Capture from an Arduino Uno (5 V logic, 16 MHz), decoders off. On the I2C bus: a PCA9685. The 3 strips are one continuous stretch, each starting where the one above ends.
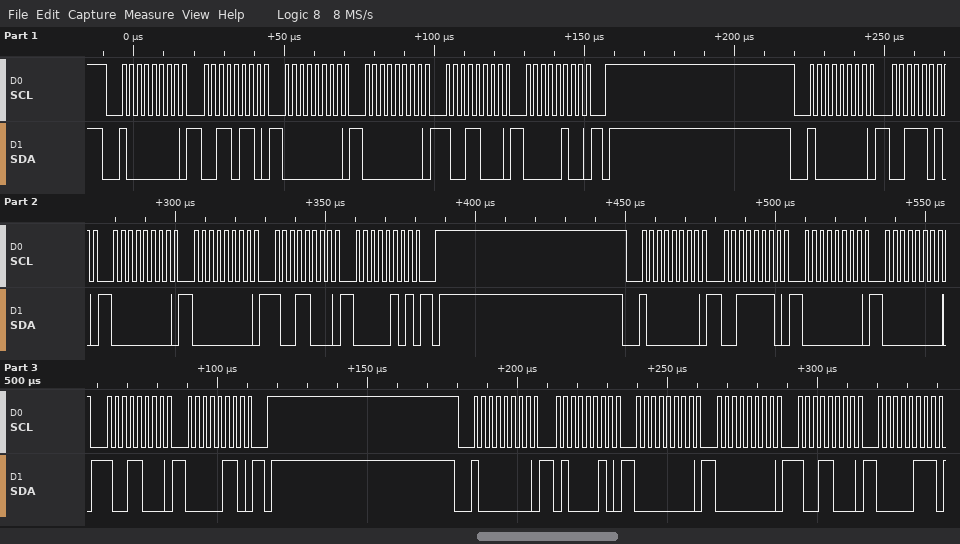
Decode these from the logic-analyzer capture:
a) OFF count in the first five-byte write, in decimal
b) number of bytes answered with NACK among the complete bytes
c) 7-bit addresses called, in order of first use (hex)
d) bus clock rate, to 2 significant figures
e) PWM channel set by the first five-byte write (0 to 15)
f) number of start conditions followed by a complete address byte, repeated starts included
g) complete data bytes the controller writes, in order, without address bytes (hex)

1176
0
0x40
400 kHz
12
4
36 00 00 98 04 3A 00 00 98 05 3E 00 00 98 06 42 00 00 98 07
